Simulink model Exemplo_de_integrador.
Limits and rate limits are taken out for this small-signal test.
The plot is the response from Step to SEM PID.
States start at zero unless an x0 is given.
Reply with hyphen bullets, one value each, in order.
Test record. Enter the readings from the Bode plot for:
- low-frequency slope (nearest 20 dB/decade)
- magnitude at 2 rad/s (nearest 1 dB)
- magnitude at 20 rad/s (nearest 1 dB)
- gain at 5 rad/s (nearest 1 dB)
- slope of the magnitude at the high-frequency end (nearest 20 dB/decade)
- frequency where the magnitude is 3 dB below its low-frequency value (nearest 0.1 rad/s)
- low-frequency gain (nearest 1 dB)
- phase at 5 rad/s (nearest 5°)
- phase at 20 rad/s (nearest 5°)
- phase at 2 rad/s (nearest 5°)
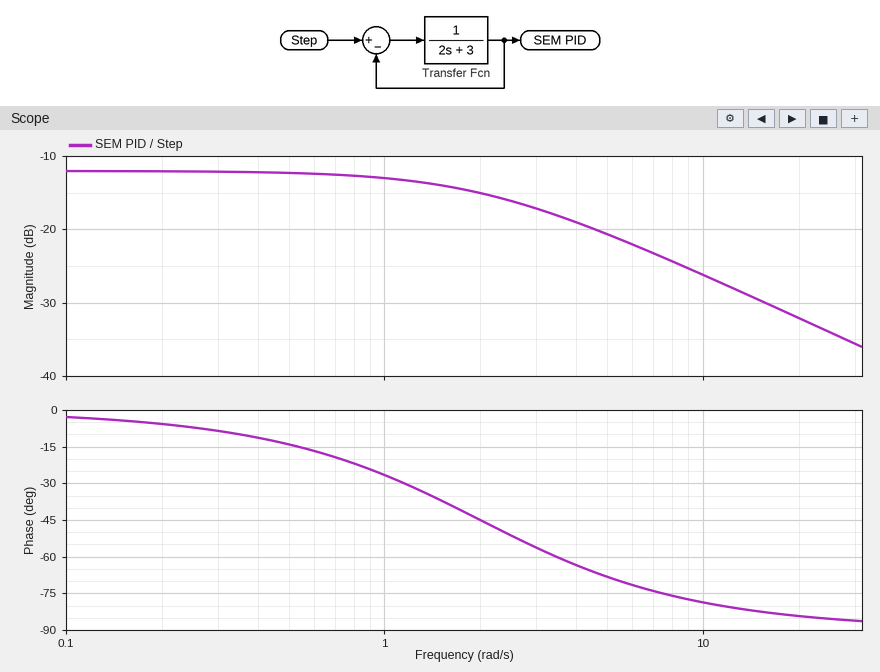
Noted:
- 0 dB/decade
- -15 dB
- -32 dB
- -21 dB
- -20 dB/decade
- 2.0 rad/s
- -12 dB
- -70°
- -85°
- -45°
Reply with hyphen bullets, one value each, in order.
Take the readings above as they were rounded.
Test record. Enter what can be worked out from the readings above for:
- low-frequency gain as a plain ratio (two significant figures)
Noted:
- 0.25
